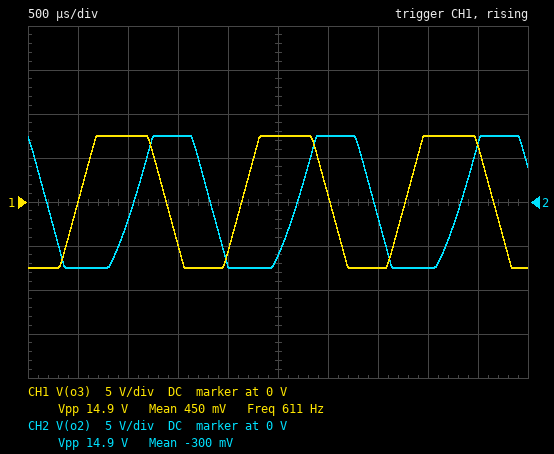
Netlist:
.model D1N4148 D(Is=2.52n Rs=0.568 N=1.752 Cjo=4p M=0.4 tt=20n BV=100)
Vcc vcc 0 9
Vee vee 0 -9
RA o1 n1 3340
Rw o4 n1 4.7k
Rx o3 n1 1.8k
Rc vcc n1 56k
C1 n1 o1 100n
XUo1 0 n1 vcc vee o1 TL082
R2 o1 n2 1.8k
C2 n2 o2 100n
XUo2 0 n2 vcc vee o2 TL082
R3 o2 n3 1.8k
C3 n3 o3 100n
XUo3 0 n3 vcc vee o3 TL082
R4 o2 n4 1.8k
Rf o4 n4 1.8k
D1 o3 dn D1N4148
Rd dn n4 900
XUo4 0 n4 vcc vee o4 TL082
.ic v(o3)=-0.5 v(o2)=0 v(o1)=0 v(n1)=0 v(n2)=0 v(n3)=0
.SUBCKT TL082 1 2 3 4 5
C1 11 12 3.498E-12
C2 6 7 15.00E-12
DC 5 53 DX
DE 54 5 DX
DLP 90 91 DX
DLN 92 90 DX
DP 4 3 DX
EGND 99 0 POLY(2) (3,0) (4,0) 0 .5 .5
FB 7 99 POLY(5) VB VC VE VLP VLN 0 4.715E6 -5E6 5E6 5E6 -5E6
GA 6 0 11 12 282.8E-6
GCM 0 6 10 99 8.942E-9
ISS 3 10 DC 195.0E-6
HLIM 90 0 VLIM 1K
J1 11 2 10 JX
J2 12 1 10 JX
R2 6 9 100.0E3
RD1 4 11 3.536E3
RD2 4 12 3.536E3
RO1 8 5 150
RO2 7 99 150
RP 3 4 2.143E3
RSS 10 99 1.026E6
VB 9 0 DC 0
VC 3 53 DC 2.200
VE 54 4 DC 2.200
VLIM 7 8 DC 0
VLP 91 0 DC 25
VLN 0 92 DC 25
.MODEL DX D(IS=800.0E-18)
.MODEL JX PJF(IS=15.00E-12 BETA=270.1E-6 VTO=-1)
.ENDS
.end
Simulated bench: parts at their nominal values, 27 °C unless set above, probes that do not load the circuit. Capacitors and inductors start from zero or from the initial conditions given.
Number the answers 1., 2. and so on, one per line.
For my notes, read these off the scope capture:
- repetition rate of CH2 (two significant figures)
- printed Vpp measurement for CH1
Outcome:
1. 610 Hz
2. 14.9 V
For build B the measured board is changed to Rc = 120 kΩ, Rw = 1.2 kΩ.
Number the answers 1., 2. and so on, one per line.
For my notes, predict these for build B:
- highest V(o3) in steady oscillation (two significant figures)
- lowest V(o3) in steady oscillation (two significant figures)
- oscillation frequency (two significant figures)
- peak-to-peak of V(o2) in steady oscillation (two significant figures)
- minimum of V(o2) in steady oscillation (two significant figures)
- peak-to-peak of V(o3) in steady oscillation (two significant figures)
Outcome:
1. 650 mV
2. -770 mV
3. 1.1 kHz
4. 1.7 V
5. -890 mV
6. 1.4 V
